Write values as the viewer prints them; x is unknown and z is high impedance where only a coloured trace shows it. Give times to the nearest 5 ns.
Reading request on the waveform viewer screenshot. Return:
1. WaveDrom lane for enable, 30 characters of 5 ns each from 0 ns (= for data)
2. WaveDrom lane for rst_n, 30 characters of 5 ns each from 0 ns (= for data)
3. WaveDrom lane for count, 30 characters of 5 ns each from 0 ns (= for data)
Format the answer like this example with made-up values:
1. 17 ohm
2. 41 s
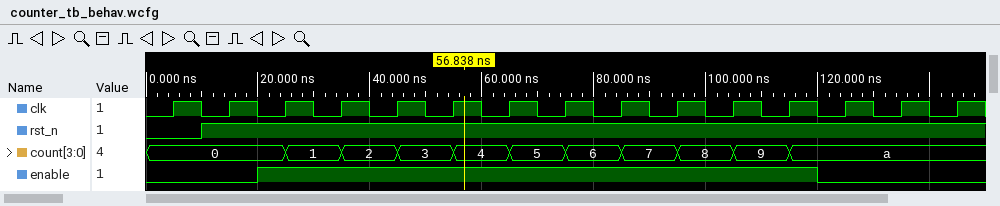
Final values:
1. {name: 'enable', wave: '0...1...................0.....'}
2. {name: 'rst_n', wave: '0.1...........................'}
3. {name: 'count', wave: '=....=.=.=.=.=.=.=.=.=.=......', data: '0 1 2 3 4 5 6 7 8 9 a'}
